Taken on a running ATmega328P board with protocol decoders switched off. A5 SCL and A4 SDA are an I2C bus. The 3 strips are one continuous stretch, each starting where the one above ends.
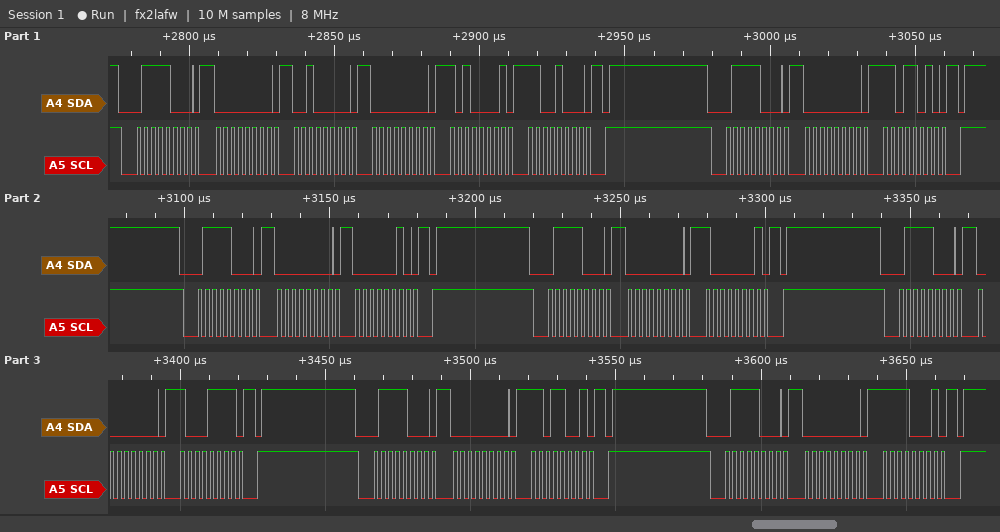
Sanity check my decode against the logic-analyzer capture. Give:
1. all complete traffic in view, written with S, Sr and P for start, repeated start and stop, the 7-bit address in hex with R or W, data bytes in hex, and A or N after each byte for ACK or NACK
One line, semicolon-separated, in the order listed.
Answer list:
S 3CW A 00 A 20 A 00 A A1 A C8 A P S 3CW A 00 A DA A P S 3CW A 00 A 02 A P S 3CW A 00 A 81 A P S 3CW A 00 A 8F A P S 3CW A 00 A D9 A P S 3CW A 00 A F1 A P
